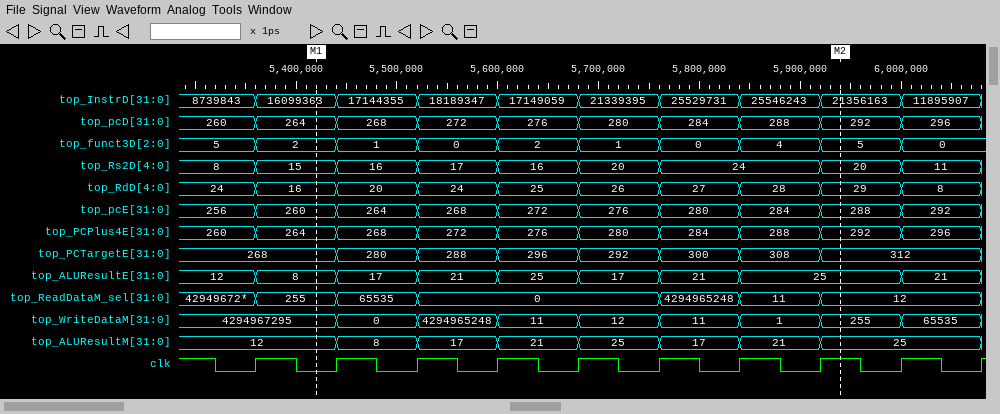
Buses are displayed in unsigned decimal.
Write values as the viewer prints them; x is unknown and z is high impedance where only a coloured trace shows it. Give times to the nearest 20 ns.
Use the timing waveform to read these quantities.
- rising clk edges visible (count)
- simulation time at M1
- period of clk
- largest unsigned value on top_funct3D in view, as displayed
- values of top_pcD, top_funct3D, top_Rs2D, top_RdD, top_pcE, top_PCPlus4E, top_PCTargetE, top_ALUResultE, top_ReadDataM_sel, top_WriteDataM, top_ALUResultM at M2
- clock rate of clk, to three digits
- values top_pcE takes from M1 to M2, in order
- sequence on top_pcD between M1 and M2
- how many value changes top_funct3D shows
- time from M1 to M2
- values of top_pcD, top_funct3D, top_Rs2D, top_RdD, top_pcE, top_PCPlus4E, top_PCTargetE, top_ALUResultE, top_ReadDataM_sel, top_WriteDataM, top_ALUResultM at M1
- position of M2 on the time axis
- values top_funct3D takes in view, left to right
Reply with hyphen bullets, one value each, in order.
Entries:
- 10
- 5420 ns
- 80 ns
- 5
- top_pcD=292, top_funct3D=5, top_Rs2D=20, top_RdD=29, top_pcE=288, top_PCPlus4E=292, top_PCTargetE=312, top_ALUResultE=25, top_ReadDataM_sel=12, top_WriteDataM=255, top_ALUResultM=25
- 12.5 MHz
- 260, 264, 268, 272, 276, 280, 284, 288
- 264, 268, 272, 276, 280, 284, 288, 292
- 9
- 520 ns
- top_pcD=264, top_funct3D=2, top_Rs2D=15, top_RdD=16, top_pcE=260, top_PCPlus4E=264, top_PCTargetE=268, top_ALUResultE=8, top_ReadDataM_sel=255, top_WriteDataM=4294967295, top_ALUResultM=12
- 5940 ns
- 5, 2, 1, 0, 2, 1, 0, 4, 5, 0
